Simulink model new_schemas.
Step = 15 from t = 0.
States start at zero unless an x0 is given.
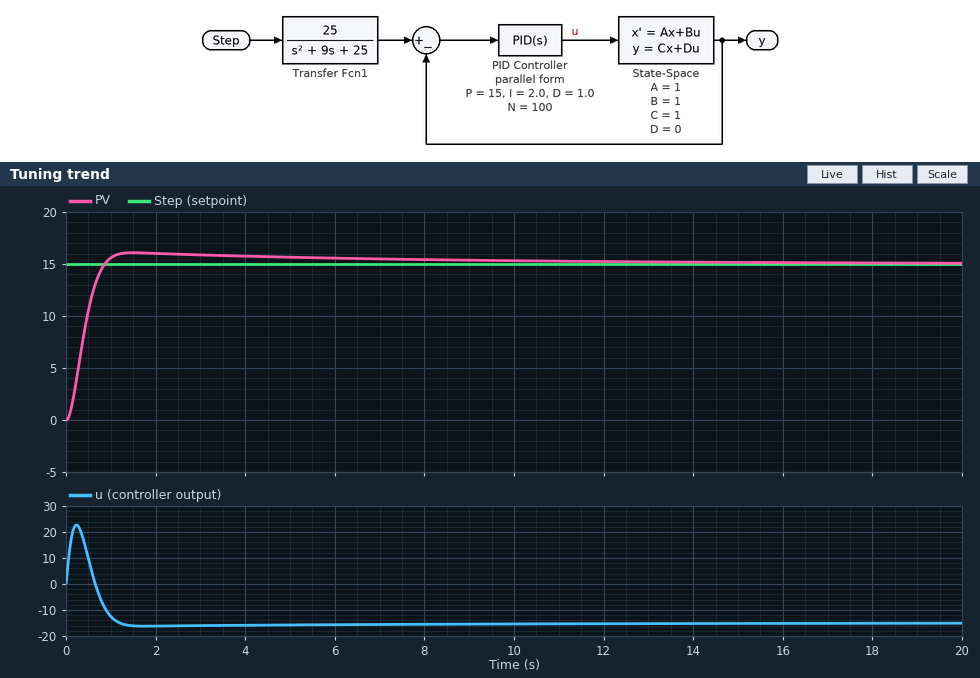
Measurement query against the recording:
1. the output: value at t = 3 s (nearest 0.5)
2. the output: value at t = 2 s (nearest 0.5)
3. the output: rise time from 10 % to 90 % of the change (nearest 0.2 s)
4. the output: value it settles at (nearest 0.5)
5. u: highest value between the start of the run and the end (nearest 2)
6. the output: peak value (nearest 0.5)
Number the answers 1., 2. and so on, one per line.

1. 16.0
2. 16.0
3. 0.6 s
4. 15.0
5. 22
6. 16.0
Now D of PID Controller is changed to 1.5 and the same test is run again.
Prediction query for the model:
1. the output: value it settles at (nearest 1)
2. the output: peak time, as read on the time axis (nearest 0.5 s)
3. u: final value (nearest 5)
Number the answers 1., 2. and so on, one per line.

1. 15
2. 1.5 s
3. -15
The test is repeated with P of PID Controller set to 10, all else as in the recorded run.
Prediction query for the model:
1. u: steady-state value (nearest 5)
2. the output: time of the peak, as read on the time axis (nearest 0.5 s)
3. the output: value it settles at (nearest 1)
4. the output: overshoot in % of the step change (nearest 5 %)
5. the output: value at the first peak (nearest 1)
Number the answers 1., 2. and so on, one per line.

1. -15
2. 1.5 s
3. 15
4. 10 %
5. 17
